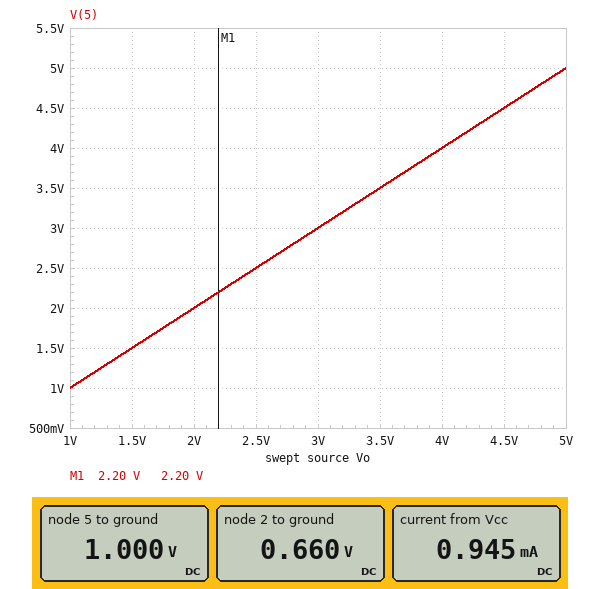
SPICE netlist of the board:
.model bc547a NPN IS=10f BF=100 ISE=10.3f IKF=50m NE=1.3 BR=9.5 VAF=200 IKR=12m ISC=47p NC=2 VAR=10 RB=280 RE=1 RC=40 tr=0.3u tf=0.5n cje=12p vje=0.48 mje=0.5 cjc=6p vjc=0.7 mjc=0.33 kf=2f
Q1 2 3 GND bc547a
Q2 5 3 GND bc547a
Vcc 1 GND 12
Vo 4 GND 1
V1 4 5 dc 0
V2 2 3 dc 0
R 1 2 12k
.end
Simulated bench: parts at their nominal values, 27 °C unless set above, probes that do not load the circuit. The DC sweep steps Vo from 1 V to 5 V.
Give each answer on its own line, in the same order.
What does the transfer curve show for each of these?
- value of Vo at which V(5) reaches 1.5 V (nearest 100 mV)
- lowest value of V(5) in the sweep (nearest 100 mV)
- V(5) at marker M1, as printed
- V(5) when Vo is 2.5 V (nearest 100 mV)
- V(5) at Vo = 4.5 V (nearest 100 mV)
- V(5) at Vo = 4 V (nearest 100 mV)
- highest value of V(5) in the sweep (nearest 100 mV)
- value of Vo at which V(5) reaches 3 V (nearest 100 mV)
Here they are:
1.5 V
1.0 V
2.20 V
2.5 V
4.5 V
4.0 V
5.0 V
3.0 V
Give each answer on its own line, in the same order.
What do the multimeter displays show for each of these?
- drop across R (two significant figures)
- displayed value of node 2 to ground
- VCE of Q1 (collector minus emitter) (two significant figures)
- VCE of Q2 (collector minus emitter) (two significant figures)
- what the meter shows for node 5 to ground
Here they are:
11 V
0.660 V
660 mV
1.0 V
1.000 V
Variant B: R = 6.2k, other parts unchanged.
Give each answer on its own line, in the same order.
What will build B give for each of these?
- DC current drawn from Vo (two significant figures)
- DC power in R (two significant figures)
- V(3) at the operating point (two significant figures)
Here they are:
1.8 mA
21 mW
680 mV
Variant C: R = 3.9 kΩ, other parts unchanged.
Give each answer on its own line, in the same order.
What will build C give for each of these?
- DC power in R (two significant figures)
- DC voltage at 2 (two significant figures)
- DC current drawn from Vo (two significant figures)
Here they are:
33 mW
700 mV
2.8 mA
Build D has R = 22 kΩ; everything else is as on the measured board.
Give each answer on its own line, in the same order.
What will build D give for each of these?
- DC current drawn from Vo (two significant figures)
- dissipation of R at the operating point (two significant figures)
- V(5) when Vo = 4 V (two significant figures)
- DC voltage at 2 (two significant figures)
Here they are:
500 µA
5.9 mW
4.0 V
640 mV
